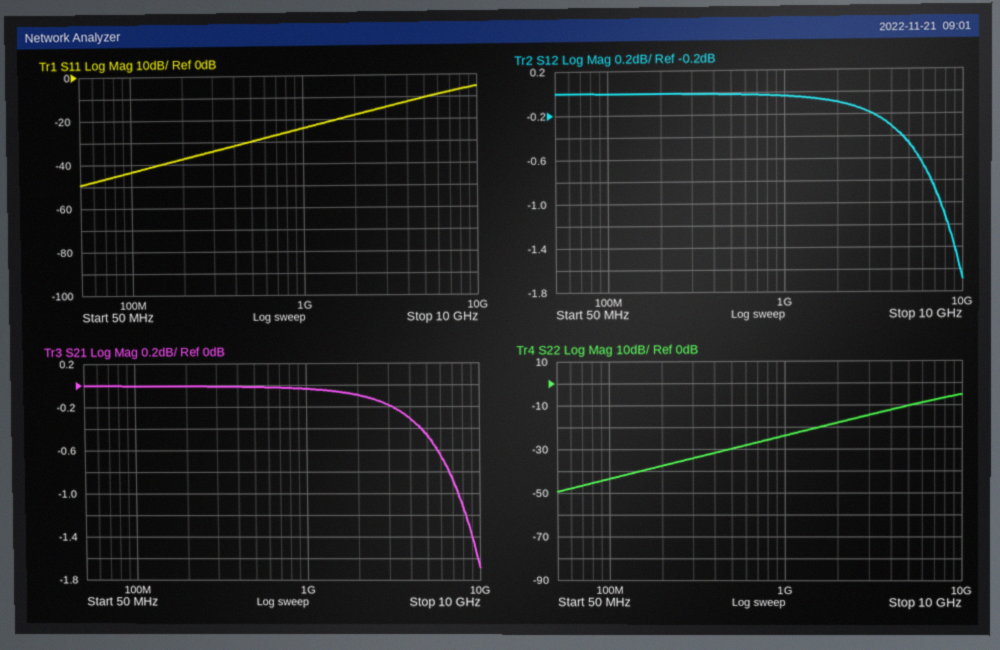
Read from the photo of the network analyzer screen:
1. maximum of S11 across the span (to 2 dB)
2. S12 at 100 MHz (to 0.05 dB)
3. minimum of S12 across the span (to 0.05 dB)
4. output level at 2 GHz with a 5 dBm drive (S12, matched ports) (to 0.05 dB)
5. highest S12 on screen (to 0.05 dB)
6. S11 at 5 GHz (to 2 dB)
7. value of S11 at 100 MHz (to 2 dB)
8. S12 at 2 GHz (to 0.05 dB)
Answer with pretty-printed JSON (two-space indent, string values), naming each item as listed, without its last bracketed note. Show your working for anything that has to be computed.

{
  "maximum of S11 across the span": "-6 dB",
  "S12 at 100 MHz": "0.00 dB",
  "minimum of S12 across the span": "-1.70 dB",
  "output level at 2 GHz with a 5 dBm drive (S12, matched ports)": "5 dBm + (-0.10 dB) = 4.90 dBm",
  "highest S12 on screen": "0.00 dB",
  "S11 at 5 GHz": "-10 dB",
  "value of S11 at 100 MHz": "-44 dB",
  "S12 at 2 GHz": "-0.10 dB"
}
